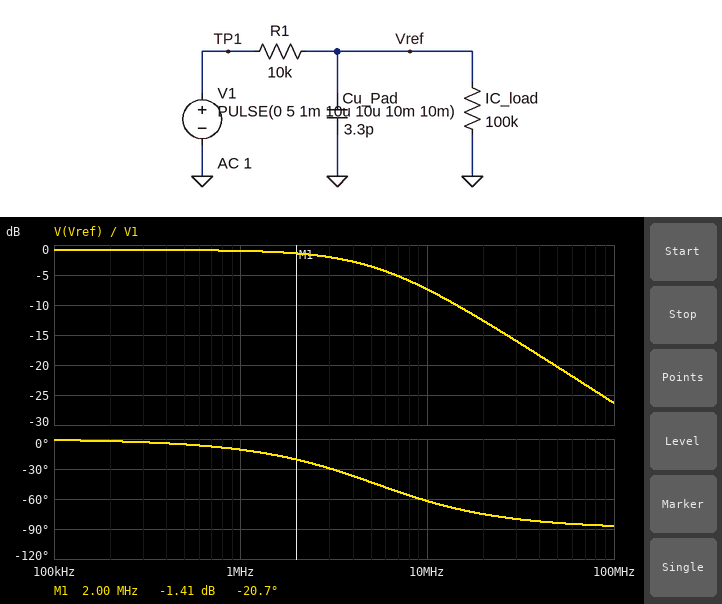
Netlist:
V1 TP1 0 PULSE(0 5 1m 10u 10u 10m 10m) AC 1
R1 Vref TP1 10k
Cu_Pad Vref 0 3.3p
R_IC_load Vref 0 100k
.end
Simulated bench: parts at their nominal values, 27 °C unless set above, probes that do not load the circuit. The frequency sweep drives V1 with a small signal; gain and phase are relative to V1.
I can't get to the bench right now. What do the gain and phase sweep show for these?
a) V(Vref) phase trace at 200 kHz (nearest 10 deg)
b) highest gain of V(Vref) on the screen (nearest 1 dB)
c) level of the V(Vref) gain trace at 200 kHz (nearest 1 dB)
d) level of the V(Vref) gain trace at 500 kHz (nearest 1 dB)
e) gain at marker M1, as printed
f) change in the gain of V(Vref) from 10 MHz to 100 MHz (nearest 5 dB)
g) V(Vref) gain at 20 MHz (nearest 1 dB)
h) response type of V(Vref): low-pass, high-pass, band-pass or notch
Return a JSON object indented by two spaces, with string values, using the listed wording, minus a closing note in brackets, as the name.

{
  "V(Vref) phase trace at 200 kHz": "0 deg",
  "highest gain of V(Vref) on the screen": "-1 dB",
  "level of the V(Vref) gain trace at 200 kHz": "-1 dB",
  "level of the V(Vref) gain trace at 500 kHz": "-1 dB",
  "gain at marker M1, as printed": "-1.41 dB",
  "change in the gain of V(Vref) from 10 MHz to 100 MHz": "-20 dB",
  "V(Vref) gain at 20 MHz": "-13 dB",
  "response type of V(Vref): low-pass, high-pass, band-pass or notch": "low-pass"
}
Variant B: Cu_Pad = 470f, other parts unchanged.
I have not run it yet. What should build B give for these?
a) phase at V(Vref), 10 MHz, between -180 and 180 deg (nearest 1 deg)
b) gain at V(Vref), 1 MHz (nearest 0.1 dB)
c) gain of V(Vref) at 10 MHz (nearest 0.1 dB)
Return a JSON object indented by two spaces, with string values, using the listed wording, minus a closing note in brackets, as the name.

{
  "phase at V(Vref), 10 MHz, between -180 and 180 deg": "-15 deg",
  "gain at V(Vref), 1 MHz": "-0.8 dB",
  "gain of V(Vref) at 10 MHz": "-1.1 dB"
}
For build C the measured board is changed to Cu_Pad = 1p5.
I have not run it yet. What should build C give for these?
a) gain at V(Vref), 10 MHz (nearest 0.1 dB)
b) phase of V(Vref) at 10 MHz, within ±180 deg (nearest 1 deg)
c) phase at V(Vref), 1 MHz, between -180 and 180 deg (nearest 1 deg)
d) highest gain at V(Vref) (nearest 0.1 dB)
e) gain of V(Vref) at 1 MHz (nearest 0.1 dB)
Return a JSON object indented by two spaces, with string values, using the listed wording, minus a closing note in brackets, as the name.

{
  "gain at V(Vref), 10 MHz": "-3.2 dB",
  "phase of V(Vref) at 10 MHz, within ±180 deg": "-41 deg",
  "phase at V(Vref), 1 MHz, between -180 and 180 deg": "-5 deg",
  "highest gain at V(Vref)": "-0.8 dB",
  "gain of V(Vref) at 1 MHz": "-0.9 dB"
}
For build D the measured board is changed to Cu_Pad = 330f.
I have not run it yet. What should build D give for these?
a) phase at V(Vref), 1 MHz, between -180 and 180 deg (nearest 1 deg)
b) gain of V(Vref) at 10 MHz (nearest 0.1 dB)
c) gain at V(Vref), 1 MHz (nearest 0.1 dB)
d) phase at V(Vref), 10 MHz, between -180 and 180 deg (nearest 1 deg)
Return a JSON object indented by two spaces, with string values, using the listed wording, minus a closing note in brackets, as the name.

{
  "phase at V(Vref), 1 MHz, between -180 and 180 deg": "-1 deg",
  "gain of V(Vref) at 10 MHz": "-1.0 dB",
  "gain at V(Vref), 1 MHz": "-0.8 dB",
  "phase at V(Vref), 10 MHz, between -180 and 180 deg": "-11 deg"
}
